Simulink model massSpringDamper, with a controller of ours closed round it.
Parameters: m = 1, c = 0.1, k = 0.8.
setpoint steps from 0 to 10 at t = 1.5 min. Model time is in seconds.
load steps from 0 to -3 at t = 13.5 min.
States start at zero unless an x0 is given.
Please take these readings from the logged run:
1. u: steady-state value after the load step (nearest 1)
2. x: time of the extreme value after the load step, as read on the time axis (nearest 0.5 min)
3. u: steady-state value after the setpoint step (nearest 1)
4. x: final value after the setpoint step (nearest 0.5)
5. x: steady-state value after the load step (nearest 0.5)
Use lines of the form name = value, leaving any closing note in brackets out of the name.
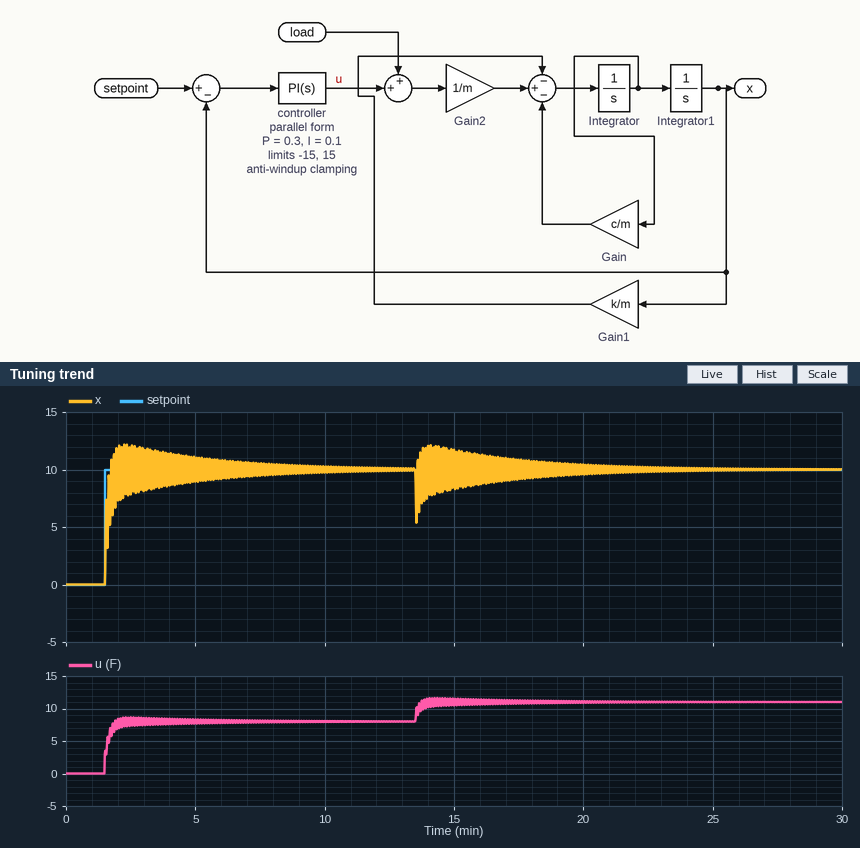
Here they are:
u: steady-state value after the load step = 11
x: time of the extreme value after the load step, as read on the time axis = 13.5 min
u: steady-state value after the setpoint step = 8
x: final value after the setpoint step = 10.0
x: steady-state value after the load step = 10.0
